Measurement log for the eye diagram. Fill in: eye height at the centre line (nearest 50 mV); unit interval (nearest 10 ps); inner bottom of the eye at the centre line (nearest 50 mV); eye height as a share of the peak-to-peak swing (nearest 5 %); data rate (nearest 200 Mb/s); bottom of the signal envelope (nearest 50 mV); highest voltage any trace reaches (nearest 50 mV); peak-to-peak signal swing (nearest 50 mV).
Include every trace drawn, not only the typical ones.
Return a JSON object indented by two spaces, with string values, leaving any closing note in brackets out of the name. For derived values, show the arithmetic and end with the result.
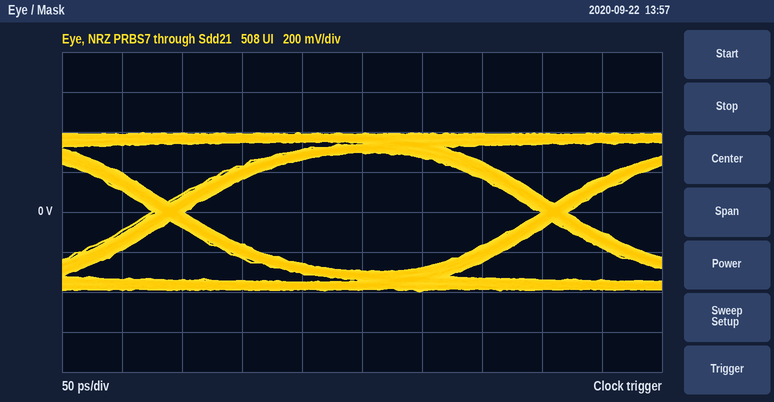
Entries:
{
  "eye height at the centre line": "600 mV",
  "unit interval": "320 ps",
  "inner bottom of the eye at the centre line": "-300 mV",
  "eye height as a share of the peak-to-peak swing": "600 mV / 800 mV ≈ 75 %",
  "data rate": "3.2 Gb/s",
  "bottom of the signal envelope": "-400 mV",
  "highest voltage any trace reaches": "400 mV",
  "peak-to-peak signal swing": "800 mV"
}
